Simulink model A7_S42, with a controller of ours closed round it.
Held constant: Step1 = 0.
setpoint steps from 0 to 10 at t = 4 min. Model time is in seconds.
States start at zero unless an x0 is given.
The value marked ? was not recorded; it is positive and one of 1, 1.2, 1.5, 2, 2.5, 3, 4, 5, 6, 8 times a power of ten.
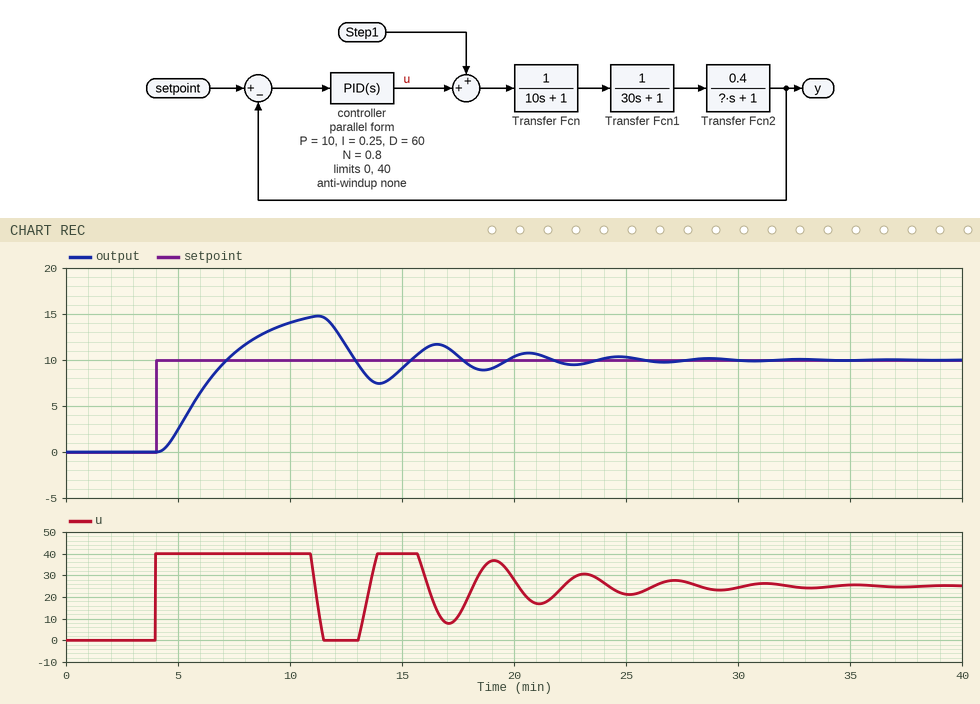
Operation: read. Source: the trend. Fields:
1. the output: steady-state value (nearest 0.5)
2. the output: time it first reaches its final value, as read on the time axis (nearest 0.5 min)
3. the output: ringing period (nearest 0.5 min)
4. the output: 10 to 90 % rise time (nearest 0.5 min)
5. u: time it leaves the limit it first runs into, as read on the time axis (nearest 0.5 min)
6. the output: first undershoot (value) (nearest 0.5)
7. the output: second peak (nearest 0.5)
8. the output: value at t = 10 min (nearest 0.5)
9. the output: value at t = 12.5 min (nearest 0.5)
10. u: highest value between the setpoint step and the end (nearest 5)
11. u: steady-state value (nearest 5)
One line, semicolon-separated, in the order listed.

10.0; 7.0 min; 5.5 min; 2.0 min; 11.0 min; 7.5; 11.5; 14.0; 11.5; 40; 25
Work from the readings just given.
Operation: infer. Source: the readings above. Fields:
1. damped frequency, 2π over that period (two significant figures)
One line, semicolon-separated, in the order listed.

1.1 rad/min
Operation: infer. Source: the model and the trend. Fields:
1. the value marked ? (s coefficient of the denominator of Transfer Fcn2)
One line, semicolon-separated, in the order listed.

150
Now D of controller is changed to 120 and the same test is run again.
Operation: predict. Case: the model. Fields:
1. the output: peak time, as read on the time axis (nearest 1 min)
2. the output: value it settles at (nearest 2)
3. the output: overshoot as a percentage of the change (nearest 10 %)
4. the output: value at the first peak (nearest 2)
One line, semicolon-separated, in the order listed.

11 min; 10; 50 %; 14
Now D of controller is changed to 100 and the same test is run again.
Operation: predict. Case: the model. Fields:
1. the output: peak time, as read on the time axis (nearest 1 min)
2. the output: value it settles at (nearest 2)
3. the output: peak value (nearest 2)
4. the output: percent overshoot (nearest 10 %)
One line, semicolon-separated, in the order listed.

11 min; 10; 14; 50 %
